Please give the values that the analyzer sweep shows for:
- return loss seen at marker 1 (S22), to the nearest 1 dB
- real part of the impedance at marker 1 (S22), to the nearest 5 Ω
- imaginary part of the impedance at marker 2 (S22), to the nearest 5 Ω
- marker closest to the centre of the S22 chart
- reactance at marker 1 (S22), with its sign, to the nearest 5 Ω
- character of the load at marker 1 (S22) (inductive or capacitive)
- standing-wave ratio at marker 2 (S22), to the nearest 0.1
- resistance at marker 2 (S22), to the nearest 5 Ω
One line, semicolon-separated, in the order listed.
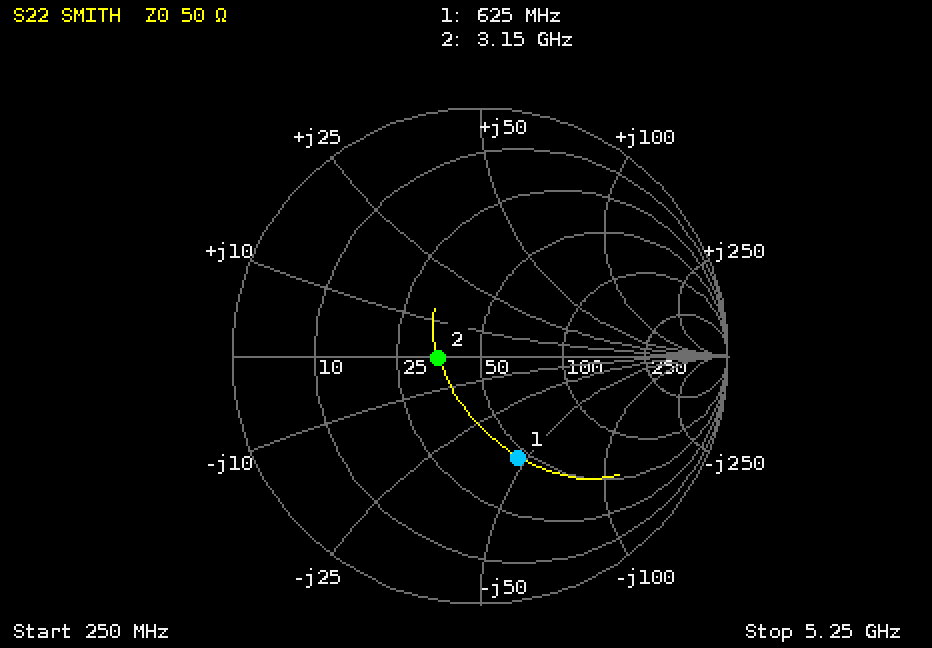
7 dB; 45 Ω; 0 Ω; marker 2; -45 Ω; capacitive; 1.4; 35 Ω
